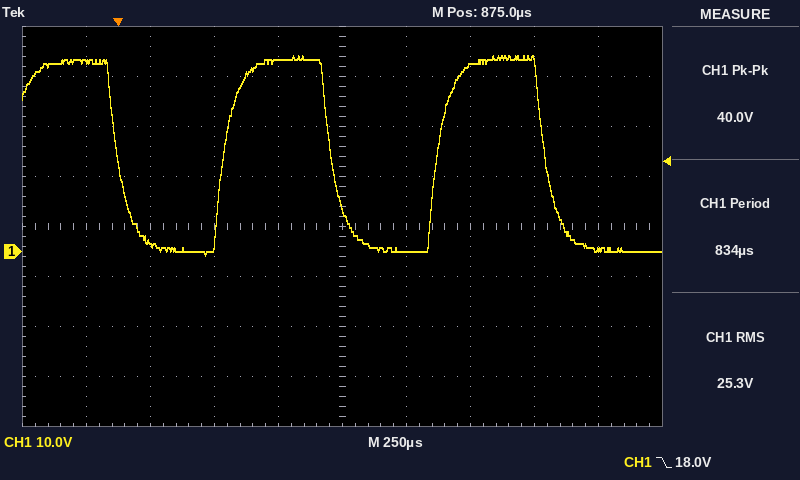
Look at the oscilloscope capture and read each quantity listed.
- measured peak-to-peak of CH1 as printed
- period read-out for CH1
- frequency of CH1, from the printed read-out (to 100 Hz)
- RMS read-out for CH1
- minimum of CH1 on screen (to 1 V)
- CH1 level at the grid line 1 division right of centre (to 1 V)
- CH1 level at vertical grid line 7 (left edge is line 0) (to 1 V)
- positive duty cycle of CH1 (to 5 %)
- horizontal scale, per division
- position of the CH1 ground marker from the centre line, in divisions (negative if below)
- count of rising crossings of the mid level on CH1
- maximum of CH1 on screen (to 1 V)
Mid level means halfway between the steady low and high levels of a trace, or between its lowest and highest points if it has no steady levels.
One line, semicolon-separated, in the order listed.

40.0 V; 834 µs; 1.2 kHz; 25.3 V; -1 V; 0 V; 37 V; 50 %; 250 µs; -0.5 div; 2; 39 V
